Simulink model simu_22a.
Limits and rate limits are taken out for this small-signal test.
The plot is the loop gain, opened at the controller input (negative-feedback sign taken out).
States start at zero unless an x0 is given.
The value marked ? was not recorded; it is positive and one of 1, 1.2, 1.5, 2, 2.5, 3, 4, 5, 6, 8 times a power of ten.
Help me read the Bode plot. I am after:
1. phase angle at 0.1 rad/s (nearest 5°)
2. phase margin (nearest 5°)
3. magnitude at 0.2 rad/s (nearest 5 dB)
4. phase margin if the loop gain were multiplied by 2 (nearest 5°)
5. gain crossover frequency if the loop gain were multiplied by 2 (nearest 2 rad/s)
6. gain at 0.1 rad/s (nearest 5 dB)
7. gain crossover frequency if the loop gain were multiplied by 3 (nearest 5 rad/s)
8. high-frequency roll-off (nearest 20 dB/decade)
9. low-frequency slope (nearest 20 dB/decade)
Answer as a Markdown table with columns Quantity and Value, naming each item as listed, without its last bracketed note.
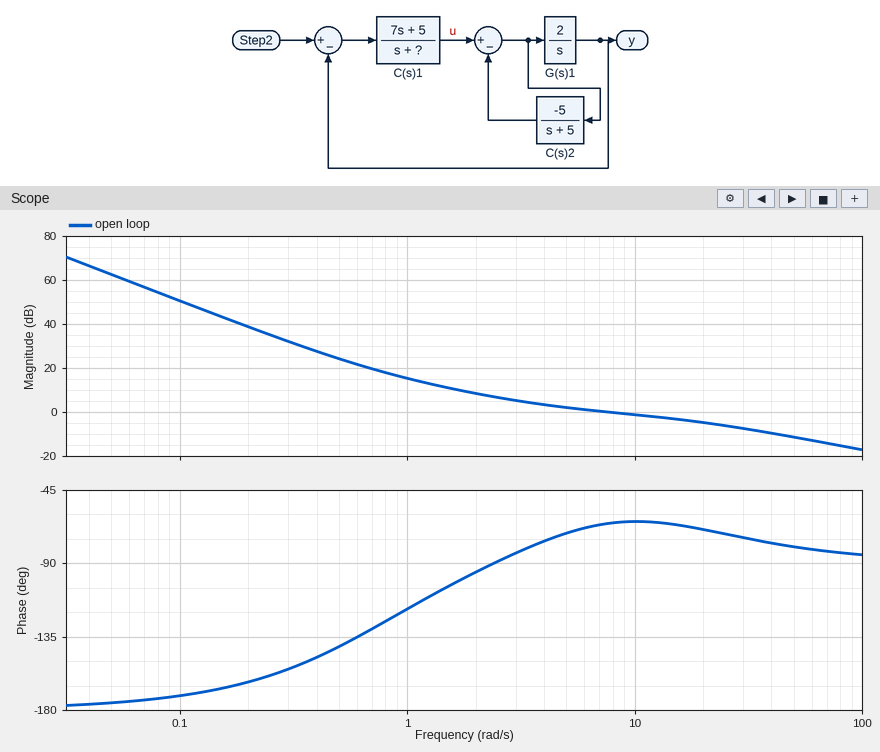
| Quantity | Value |
|---|---|
| phase angle at 0.1 rad/s | -170° |
| phase margin | 115° |
| magnitude at 0.2 rad/s | 40 dB |
| phase margin if the loop gain were multiplied by 2 | 110° |
| gain crossover frequency if the loop gain were multiplied by 2 | 24 rad/s |
| gain at 0.1 rad/s | 50 dB |
| gain crossover frequency if the loop gain were multiplied by 3 | 40 rad/s |
| high-frequency roll-off | -20 dB/decade |
| low-frequency slope | -40 dB/decade |
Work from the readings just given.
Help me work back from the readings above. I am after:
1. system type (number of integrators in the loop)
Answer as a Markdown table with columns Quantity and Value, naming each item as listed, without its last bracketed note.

| Quantity | Value |
|---|---|
| system type | 2 |
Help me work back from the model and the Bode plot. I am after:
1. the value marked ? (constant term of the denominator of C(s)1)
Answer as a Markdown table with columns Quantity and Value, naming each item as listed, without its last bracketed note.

| Quantity | Value |
|---|---|
| the value marked ? (constant term of the denominator of C(s)1) | 15 |
